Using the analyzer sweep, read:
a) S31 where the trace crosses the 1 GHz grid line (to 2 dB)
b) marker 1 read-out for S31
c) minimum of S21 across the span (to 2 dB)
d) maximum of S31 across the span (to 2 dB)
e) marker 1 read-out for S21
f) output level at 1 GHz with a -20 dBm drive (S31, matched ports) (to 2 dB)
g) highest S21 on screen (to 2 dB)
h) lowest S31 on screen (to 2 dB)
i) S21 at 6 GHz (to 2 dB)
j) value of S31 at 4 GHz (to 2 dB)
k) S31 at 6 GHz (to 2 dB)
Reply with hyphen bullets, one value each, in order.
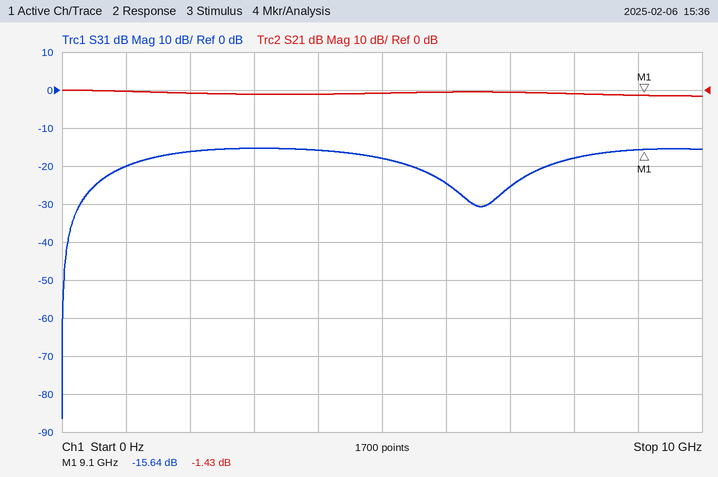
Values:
- -20 dB
- -15.64 dB
- -2 dB
- -16 dB
- -1.43 dB
- -40 dBm
- 0 dB
- -86 dB
- 0 dB
- -16 dB
- -24 dB
